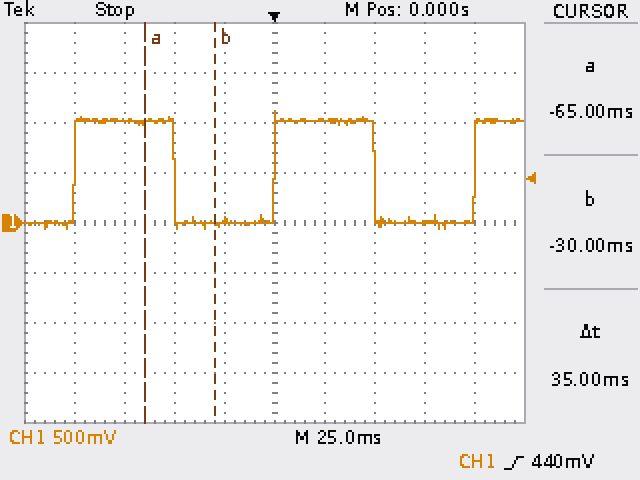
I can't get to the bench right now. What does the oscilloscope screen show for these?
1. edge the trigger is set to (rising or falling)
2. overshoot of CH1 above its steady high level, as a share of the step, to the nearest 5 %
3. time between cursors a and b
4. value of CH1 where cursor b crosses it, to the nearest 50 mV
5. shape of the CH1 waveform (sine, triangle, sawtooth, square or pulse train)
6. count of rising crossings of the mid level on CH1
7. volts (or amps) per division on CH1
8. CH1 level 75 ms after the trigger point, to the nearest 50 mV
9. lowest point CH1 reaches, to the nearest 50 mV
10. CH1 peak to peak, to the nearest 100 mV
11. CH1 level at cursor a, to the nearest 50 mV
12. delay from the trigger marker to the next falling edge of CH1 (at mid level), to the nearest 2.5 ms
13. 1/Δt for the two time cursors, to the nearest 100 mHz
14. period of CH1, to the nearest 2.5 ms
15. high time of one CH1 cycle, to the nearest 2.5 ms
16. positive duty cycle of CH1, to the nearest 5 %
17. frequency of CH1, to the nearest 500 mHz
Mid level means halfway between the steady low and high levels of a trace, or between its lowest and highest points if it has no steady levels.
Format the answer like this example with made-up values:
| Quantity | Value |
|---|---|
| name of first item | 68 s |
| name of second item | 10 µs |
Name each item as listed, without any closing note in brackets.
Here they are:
| Quantity | Value |
|---|---|
| edge the trigger is set to | rising |
| overshoot of CH1 above its steady high level, as a share of the step, to the nearest 5 % | 10 % |
| time between cursors a and b | 35 ms |
| value of CH1 where cursor b crosses it, to the nearest 50 mV | 0 mV |
| shape of the CH1 waveform | square |
| count of rising crossings of the mid level on CH1 | 3 |
| volts (or amps) per division on CH1 | 500 mV |
| CH1 level 75 ms after the trigger point, to the nearest 50 mV | 0 mV |
| lowest point CH1 reaches, to the nearest 50 mV | -50 mV |
| CH1 peak to peak, to the nearest 100 mV | 1.20 V |
| CH1 level at cursor a, to the nearest 50 mV | 1.00 V |
| delay from the trigger marker to the next falling edge of CH1 (at mid level), to the nearest 2.5 ms | 50.0 ms |
| 1/Δt for the two time cursors, to the nearest 100 mHz | 28.6 Hz |
| period of CH1, to the nearest 2.5 ms | 100.0 ms |
| high time of one CH1 cycle, to the nearest 2.5 ms | 50.0 ms |
| positive duty cycle of CH1, to the nearest 5 % | 50 % |
| frequency of CH1, to the nearest 500 mHz | 10.0 Hz |
